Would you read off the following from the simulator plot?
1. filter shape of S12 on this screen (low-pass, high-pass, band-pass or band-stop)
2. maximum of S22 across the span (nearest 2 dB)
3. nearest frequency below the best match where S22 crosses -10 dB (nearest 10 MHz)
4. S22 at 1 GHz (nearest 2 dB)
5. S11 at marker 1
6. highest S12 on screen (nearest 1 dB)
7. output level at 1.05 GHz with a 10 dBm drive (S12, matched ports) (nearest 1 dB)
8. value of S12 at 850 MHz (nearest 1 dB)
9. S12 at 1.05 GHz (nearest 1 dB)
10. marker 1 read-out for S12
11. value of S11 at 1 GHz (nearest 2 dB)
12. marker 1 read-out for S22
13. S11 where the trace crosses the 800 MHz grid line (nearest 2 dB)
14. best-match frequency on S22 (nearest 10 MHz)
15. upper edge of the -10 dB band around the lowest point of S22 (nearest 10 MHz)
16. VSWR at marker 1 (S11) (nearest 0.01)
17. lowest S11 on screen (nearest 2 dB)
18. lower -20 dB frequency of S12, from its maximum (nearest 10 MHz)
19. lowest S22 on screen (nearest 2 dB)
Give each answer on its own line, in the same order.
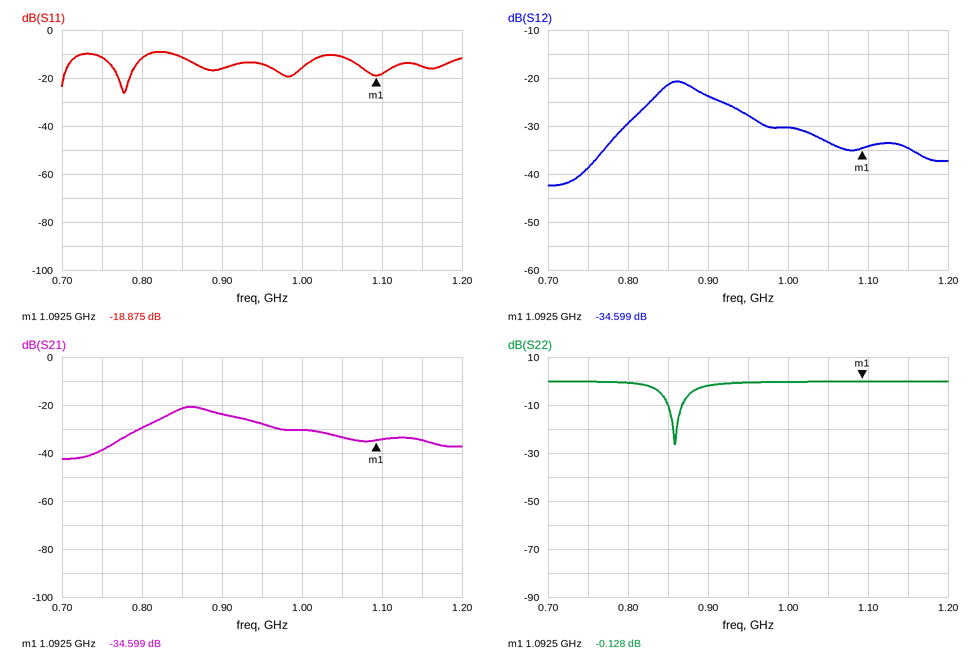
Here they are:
band-pass
0 dB
850 MHz
0 dB
-18.875 dB
-21 dB
-23 dBm
-21 dB
-33 dB
-34.599 dB
-16 dB
-0.128 dB
-12 dB
860 MHz
870 MHz
1.26
-26 dB
740 MHz
-26 dB
